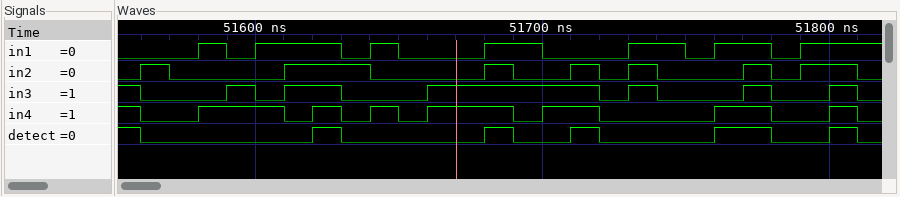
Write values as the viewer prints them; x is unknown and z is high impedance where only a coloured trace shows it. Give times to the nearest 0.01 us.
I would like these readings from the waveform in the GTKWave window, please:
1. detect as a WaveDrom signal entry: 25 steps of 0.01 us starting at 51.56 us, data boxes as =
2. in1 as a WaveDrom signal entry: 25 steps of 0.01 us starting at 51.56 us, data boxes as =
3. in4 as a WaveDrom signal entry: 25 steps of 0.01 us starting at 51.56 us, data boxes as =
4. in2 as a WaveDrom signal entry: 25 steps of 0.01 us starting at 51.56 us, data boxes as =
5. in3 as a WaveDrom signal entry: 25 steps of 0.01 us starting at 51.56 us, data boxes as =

{name: 'detect', wave: '0.....10....10.10...1.0.1'}
{name: 'in1', wave: '0.101..010..1.0..1.01.01.'}
{name: 'in4', wave: '0.1..010101..01.0...1.0.1'}
{name: 'in2', wave: '10...1..0...10.1010..101.'}
{name: 'in3', wave: '0..101.0..1.....010..10.1'}
